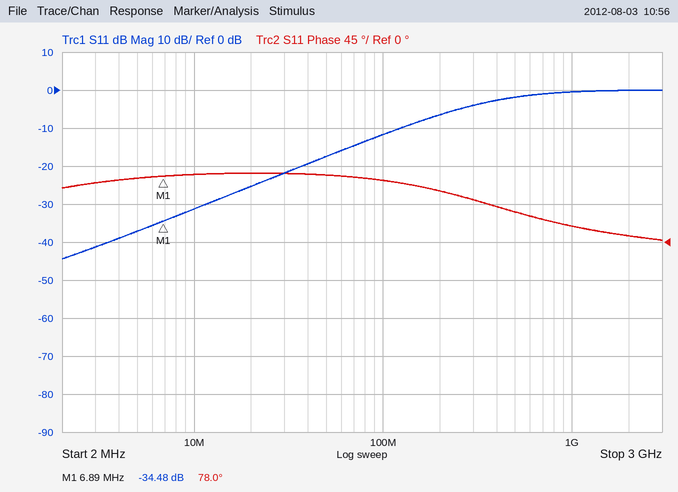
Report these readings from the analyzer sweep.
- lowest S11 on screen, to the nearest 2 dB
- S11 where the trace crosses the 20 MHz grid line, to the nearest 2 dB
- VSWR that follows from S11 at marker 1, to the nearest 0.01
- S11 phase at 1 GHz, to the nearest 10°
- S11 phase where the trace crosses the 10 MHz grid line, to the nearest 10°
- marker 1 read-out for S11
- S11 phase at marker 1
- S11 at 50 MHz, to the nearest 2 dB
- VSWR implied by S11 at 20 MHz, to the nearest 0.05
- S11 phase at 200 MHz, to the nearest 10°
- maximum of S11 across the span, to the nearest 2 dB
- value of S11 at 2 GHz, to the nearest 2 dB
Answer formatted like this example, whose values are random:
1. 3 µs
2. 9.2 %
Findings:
1. -44 dB
2. -26 dB
3. 1.04
4. 20°
5. 80°
6. -34.48 dB
7. 78.0°
8. -18 dB
9. 1.10
10. 60°
11. 0 dB
12. 0 dB
